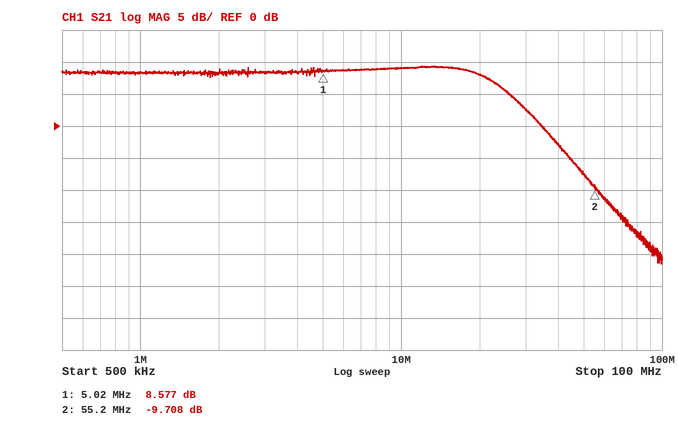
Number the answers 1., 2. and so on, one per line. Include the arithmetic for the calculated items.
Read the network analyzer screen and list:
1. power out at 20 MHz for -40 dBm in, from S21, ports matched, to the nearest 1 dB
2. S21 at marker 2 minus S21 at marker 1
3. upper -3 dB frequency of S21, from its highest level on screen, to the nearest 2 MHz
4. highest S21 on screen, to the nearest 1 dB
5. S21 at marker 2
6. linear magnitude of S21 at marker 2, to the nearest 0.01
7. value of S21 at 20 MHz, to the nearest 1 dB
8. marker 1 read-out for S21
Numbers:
1. -40 dBm + (8 dB) = -32 dBm
2. -9.708 − (8.577) = -18.285 dB
3. 24 MHz
4. 9 dB
5. -9.708 dB
6. 10^(-9.708/20) ≈ 0.33
7. 8 dB
8. 8.577 dB
